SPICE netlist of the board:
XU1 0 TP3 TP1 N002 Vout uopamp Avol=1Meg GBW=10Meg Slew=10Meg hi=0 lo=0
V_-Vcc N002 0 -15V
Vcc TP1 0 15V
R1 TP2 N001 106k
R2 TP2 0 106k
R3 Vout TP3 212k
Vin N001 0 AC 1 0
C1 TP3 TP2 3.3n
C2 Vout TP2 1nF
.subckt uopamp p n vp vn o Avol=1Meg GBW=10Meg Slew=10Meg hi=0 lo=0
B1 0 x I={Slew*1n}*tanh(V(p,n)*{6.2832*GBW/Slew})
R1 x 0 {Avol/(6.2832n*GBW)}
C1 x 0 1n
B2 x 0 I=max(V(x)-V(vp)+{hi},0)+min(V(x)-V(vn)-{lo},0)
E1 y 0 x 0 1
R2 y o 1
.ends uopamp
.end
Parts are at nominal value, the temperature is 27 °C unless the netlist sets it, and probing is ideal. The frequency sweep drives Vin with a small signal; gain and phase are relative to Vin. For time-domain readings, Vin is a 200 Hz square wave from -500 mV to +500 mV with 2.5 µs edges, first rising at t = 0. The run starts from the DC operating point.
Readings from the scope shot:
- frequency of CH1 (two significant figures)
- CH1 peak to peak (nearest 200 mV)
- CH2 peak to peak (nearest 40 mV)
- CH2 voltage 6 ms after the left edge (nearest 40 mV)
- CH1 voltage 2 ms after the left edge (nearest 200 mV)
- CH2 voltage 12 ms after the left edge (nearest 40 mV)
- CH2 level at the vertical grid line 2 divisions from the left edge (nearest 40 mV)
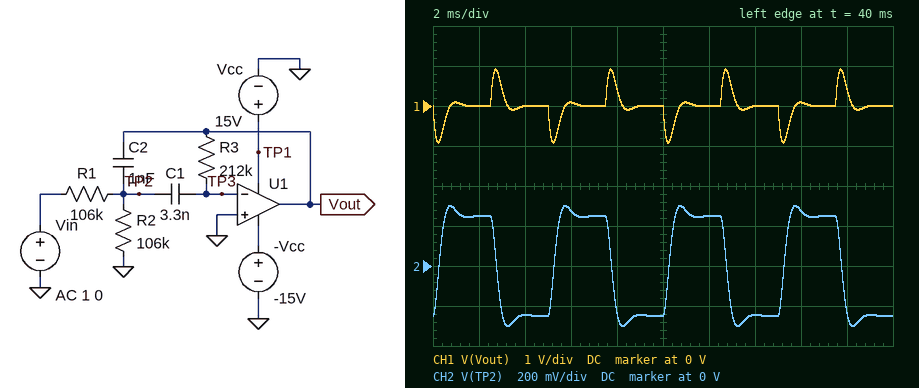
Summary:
200 Hz
1.8 V
600 mV
280 mV
0 V
240 mV
-240 mV
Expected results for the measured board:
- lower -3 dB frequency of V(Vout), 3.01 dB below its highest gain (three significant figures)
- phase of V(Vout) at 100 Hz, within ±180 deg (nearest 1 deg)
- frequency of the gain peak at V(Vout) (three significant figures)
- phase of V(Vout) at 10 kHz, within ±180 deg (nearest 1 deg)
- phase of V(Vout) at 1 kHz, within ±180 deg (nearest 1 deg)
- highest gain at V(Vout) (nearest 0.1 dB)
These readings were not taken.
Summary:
471 Hz
-98 deg
826 Hz
96 deg
162 deg
3.7 dB
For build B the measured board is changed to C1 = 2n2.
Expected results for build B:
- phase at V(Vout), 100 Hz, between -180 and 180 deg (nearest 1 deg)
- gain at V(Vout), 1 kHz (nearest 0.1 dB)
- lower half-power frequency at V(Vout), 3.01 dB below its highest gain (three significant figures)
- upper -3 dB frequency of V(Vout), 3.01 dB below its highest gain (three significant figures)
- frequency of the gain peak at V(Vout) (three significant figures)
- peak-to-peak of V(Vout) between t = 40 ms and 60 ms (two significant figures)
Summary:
-96 deg
2.8 dB
604 Hz
1.70 kHz
1.01 kHz
1.6 V
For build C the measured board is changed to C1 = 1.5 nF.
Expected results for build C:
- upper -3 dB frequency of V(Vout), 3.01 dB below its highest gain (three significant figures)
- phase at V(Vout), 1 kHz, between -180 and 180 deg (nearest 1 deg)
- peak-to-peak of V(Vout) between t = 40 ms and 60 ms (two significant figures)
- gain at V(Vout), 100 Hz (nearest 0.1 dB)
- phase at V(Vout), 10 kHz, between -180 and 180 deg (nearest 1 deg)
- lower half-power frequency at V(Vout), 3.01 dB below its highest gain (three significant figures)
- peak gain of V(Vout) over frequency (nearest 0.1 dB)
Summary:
2.00 kHz
-158 deg
1.3 V
-20.0 dB
97 deg
751 Hz
1.6 dB
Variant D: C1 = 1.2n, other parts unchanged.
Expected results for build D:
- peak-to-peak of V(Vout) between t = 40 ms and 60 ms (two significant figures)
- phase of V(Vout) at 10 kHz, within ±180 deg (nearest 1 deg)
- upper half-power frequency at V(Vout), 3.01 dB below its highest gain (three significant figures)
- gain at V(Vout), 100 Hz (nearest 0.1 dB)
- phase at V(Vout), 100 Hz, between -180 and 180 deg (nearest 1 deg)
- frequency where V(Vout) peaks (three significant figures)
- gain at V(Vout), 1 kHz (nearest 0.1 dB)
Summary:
1.2 V
98 deg
2.22 kHz
-21.9 dB
-94 deg
1.37 kHz
-0.7 dB
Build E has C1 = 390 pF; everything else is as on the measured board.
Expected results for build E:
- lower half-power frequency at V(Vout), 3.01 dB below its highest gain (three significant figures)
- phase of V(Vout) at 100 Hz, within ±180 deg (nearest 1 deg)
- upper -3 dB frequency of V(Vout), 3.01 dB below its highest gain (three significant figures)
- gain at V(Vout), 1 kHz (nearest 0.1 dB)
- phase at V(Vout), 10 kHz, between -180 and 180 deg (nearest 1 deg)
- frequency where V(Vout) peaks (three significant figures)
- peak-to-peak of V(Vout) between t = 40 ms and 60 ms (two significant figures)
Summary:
1.41 kHz
-93 deg
4.09 kHz
-11.2 dB
106 deg
2.40 kHz
650 mV
